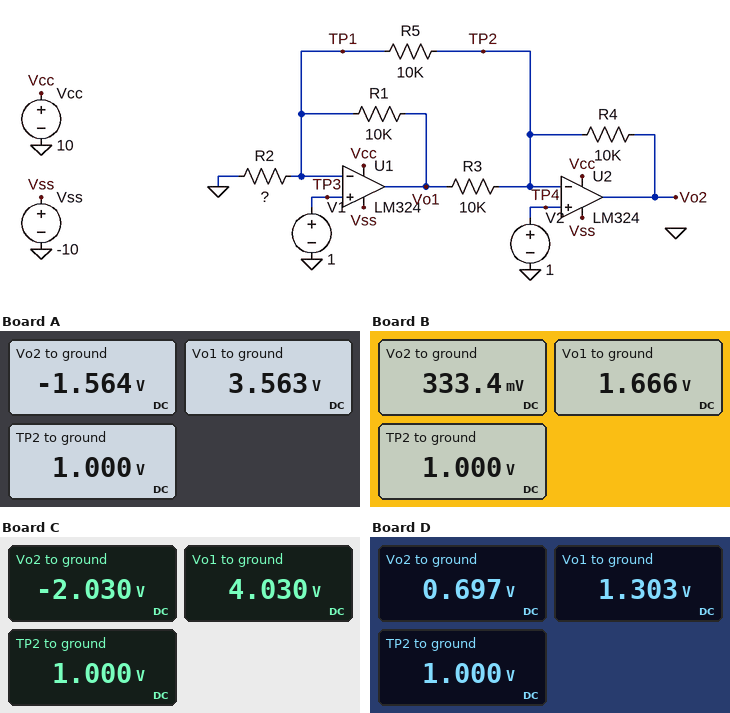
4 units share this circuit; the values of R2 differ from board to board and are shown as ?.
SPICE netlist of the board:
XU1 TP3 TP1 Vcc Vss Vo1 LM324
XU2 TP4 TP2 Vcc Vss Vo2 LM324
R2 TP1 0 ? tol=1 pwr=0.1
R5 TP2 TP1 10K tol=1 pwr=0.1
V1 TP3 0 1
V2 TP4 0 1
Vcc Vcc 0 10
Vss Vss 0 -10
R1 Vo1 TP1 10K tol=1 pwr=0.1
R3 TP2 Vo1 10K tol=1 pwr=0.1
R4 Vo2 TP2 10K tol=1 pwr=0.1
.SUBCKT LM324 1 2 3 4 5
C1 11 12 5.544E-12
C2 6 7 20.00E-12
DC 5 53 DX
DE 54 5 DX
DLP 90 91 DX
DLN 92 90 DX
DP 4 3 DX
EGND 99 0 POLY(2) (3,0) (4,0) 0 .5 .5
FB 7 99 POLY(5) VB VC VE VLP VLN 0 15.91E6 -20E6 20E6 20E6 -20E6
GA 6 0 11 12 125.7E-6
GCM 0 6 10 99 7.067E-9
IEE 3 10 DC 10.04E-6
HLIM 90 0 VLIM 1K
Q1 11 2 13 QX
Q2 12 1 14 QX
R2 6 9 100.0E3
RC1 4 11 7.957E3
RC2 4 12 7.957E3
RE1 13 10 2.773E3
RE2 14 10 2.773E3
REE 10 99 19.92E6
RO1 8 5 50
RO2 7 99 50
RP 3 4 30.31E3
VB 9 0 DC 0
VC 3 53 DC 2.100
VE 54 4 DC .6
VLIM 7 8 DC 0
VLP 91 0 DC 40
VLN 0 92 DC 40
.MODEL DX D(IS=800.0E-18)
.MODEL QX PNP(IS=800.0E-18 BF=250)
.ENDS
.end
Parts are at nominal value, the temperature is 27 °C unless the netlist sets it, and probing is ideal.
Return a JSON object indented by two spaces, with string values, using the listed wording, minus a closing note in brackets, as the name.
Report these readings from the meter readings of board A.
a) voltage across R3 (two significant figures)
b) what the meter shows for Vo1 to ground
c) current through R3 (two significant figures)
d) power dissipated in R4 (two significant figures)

{
  "voltage across R3": "2.6 V",
  "what the meter shows for Vo1 to ground": "3.563 V",
  "current through R3": "260 µA",
  "power dissipated in R4": "660 µW"
}
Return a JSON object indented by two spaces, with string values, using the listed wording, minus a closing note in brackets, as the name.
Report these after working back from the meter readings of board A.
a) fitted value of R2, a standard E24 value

{
  "fitted value of R2, a standard E24 value": "3.9 kΩ"
}
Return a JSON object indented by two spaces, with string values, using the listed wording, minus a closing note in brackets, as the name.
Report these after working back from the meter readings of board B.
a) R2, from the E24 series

{
  "R2, from the E24 series": "15 kΩ"
}
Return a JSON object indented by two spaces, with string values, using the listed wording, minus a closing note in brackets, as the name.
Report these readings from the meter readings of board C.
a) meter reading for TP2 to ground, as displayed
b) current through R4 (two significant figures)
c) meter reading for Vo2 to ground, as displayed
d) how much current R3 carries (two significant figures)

{
  "meter reading for TP2 to ground, as displayed": "1.000 V",
  "current through R4": "300 µA",
  "meter reading for Vo2 to ground, as displayed": "-2.030 V",
  "how much current R3 carries": "300 µA"
}
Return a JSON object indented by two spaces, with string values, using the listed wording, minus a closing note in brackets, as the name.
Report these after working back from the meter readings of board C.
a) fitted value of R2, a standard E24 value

{
  "fitted value of R2, a standard E24 value": "3.3 kΩ"
}
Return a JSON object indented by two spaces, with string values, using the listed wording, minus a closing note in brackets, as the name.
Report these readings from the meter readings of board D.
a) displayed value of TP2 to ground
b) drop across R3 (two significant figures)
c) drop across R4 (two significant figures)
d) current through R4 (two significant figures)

{
  "displayed value of TP2 to ground": "1.000 V",
  "drop across R3": "300 mV",
  "drop across R4": "300 mV",
  "current through R4": "30 µA"
}
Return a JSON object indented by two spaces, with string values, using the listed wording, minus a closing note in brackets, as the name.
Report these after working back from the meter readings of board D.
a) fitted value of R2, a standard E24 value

{
  "fitted value of R2, a standard E24 value": "33 kΩ"
}
